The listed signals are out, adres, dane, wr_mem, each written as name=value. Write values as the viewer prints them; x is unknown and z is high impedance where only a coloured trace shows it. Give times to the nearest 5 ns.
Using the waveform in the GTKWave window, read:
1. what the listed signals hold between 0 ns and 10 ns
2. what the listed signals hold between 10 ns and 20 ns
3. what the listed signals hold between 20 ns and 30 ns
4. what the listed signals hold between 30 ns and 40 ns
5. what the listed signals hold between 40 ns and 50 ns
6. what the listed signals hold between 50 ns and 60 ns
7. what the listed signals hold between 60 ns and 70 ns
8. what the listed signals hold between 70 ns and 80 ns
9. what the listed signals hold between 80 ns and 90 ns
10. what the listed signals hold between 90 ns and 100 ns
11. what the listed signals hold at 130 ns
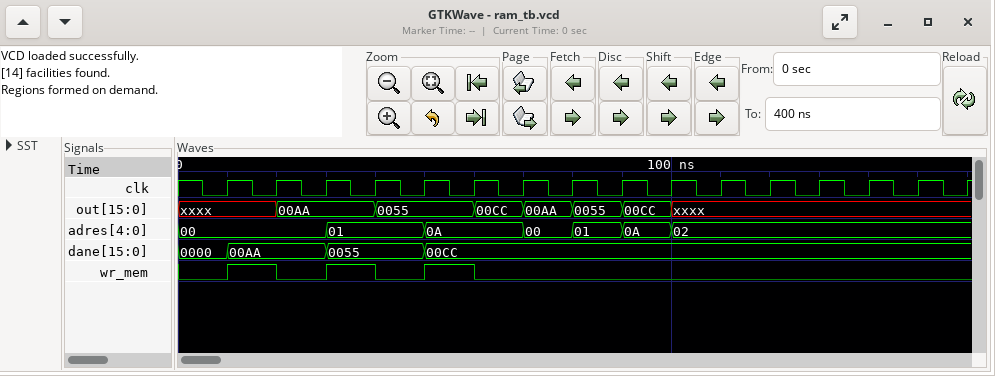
out=xxxx, adres=00, dane=0000, wr_mem=0
out=xxxx, adres=00, dane=00AA, wr_mem=1
out=00AA, adres=00, dane=00AA, wr_mem=0
out=00AA, adres=01, dane=0055, wr_mem=1
out=0055, adres=01, dane=0055, wr_mem=0
out=0055, adres=0A, dane=00CC, wr_mem=1
out=00CC, adres=0A, dane=00CC, wr_mem=0
out=00AA, adres=00, dane=00CC, wr_mem=0
out=0055, adres=01, dane=00CC, wr_mem=0
out=00CC, adres=0A, dane=00CC, wr_mem=0
out=xxxx, adres=02, dane=00CC, wr_mem=0
